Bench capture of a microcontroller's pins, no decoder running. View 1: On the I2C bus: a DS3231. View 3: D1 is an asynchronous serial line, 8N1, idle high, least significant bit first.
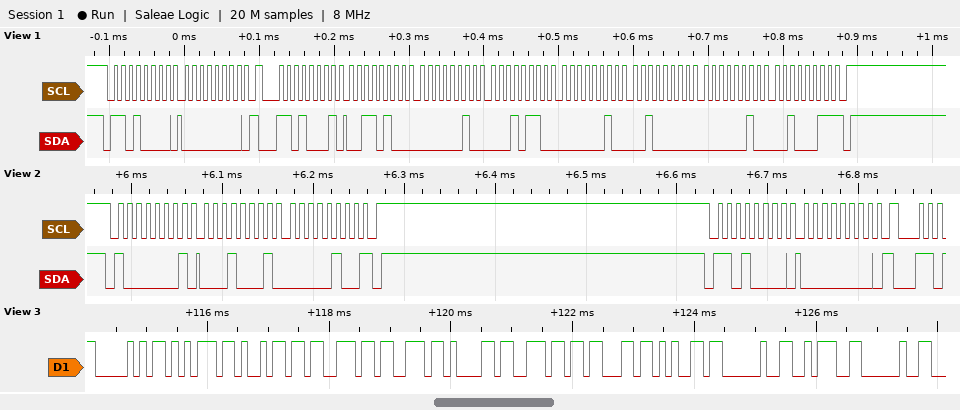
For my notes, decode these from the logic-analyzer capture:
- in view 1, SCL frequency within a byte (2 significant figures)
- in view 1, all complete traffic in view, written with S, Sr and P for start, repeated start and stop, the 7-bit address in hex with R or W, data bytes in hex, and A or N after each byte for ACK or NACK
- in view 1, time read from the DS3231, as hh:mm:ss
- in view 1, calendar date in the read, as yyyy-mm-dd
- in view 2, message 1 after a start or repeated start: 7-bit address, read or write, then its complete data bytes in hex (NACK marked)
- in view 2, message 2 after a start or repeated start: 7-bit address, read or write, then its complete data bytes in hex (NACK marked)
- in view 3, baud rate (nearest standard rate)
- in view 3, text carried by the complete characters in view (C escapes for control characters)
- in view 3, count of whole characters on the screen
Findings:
100 kHz
S 68W A 00 A Sr 68R A 34 A 02 A 16 A 02 A 20 A 02 A 23 N P
16:02:34
2023-02-20
0x40 read: 11 04 NACK
0x68 write: 00
9600 baud
"Puissance : "
12
